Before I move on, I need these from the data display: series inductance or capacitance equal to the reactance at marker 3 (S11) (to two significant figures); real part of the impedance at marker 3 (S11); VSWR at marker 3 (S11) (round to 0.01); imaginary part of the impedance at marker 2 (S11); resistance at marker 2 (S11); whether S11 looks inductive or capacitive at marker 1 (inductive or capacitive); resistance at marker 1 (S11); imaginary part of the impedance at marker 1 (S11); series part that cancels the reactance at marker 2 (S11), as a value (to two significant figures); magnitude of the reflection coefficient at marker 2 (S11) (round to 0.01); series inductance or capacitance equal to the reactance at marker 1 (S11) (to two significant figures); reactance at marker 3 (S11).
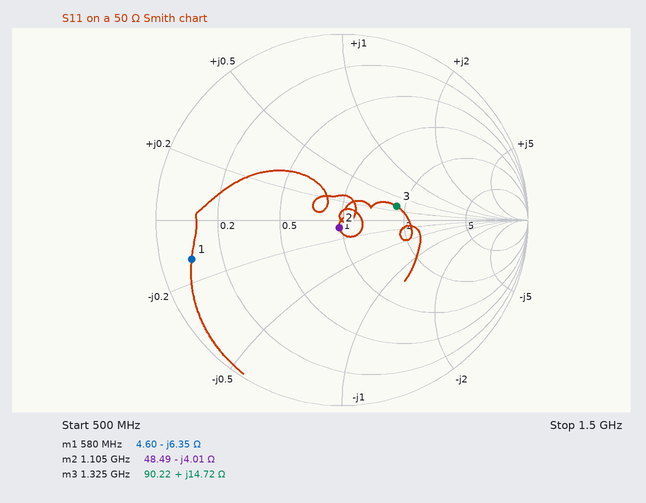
1.8 nH
90.22 Ω
1.87
-4.01 Ω
48.49 Ω
capacitive
4.60 Ω
-6.35 Ω
580 pH
0.04
43 pF
+14.72 Ω
